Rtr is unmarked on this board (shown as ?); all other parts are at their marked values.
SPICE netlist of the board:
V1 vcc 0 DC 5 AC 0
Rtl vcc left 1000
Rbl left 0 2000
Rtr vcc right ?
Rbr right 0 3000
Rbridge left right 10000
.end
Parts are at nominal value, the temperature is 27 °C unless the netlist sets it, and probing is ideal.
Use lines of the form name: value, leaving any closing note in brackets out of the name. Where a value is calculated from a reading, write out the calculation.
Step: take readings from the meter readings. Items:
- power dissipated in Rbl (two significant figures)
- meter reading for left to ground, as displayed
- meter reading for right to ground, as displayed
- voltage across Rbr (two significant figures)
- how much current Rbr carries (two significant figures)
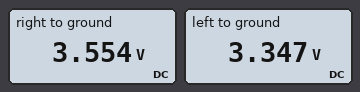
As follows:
power dissipated in Rbl: (3.347 V)^2 / 2 kΩ = 5.6 mW
meter reading for left to ground, as displayed: 3.347 V
meter reading for right to ground, as displayed: 3.554 V
voltage across Rbr: 3.554 V = 3.6 V
how much current Rbr carries: (3.554 V) / 3 kΩ = 1.2 mA
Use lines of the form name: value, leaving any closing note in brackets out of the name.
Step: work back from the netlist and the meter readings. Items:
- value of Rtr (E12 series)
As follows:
value of Rtr: 1.2 kΩ
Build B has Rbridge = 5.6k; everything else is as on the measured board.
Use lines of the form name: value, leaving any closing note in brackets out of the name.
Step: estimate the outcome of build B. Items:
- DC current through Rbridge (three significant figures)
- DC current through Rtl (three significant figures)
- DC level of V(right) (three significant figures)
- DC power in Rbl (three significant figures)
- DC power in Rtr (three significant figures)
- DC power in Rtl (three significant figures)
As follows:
DC current through Rbridge: 33.4 µA
DC current through Rtl: 1.64 mA
DC level of V(right): 3.54 V
DC power in Rbl: 5.63 mW
DC power in Rtr: 1.77 mW
DC power in Rtl: 2.70 mW
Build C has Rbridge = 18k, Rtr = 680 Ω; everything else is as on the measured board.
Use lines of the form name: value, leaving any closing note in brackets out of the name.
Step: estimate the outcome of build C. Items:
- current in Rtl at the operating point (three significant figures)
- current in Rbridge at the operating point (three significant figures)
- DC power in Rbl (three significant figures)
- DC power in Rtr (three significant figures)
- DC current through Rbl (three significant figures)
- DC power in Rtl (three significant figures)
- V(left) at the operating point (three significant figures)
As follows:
current in Rtl at the operating point: 1.64 mA
current in Rbridge at the operating point: 38.6 µA
DC power in Rbl: 5.64 mW
DC power in Rtr: 1.31 mW
DC current through Rbl: 1.68 mA
DC power in Rtl: 2.69 mW
V(left) at the operating point: 3.36 V
